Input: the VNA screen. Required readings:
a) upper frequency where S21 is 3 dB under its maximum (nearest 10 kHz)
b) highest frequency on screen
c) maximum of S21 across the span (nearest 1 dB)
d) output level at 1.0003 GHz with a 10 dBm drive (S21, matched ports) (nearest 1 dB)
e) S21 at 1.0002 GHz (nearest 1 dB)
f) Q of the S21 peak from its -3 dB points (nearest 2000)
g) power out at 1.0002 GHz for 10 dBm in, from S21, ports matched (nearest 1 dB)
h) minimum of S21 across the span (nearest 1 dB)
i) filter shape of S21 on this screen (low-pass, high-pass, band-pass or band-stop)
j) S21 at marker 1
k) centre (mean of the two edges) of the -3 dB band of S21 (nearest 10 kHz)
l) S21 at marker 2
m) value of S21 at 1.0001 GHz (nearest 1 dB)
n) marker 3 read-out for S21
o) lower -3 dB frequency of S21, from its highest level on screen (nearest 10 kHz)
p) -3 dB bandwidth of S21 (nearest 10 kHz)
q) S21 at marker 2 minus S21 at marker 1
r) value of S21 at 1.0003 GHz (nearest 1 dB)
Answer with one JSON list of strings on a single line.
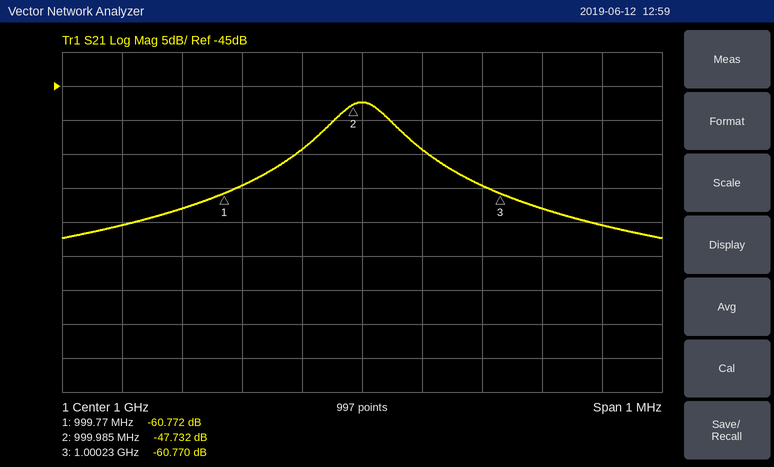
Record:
["1.00005 GHz", "1.0005 GHz", "-47 dB", "-53 dBm", "-60 dB", "10000", "-50 dBm", "-67 dB", "band-pass", "-60.772 dB", "1.00000 GHz", "-47.732 dB", "-54 dB", "-60.770 dB", "999.95 MHz", "100 kHz", "13.040 dB", "-63 dB"]
